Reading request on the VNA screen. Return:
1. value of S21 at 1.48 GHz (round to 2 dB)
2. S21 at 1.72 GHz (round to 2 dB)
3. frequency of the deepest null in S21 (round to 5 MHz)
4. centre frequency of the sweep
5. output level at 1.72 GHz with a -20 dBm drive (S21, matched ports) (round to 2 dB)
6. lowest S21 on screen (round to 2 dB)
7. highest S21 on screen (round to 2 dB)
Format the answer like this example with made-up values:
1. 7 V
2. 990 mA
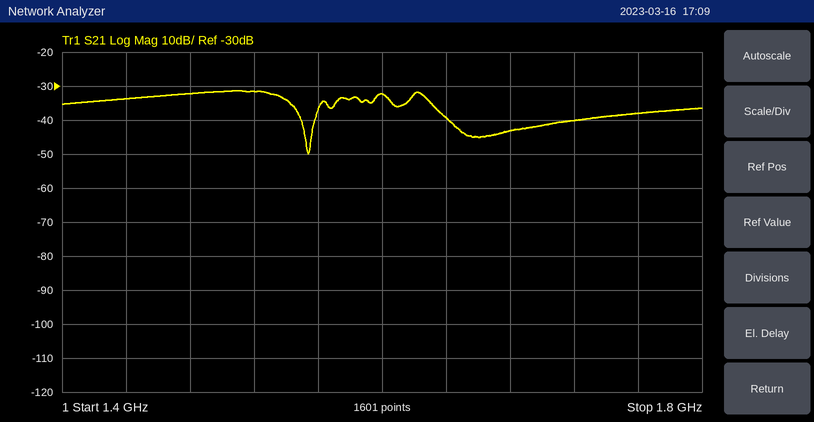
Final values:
1. -32 dB
2. -40 dB
3. 1.555 GHz
4. 1.6 GHz
5. -60 dBm
6. -50 dB
7. -32 dB
